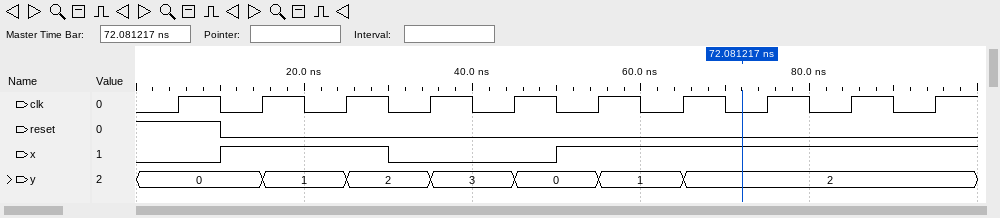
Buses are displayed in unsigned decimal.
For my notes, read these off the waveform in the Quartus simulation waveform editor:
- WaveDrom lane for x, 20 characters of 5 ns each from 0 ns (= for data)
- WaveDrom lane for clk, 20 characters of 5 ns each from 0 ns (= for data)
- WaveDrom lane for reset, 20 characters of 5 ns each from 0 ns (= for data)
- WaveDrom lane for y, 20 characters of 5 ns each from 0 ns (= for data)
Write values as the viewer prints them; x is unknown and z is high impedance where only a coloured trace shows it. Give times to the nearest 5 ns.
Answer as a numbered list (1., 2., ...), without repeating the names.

1. {name: 'x', wave: '0.1...0...1.........'}
2. {name: 'clk', wave: '01010101010101010101'}
3. {name: 'reset', wave: '1.0.................'}
4. {name: 'y', wave: '=..=.=.=.=.=.=......', data: '0 1 2 3 0 1 2'}
